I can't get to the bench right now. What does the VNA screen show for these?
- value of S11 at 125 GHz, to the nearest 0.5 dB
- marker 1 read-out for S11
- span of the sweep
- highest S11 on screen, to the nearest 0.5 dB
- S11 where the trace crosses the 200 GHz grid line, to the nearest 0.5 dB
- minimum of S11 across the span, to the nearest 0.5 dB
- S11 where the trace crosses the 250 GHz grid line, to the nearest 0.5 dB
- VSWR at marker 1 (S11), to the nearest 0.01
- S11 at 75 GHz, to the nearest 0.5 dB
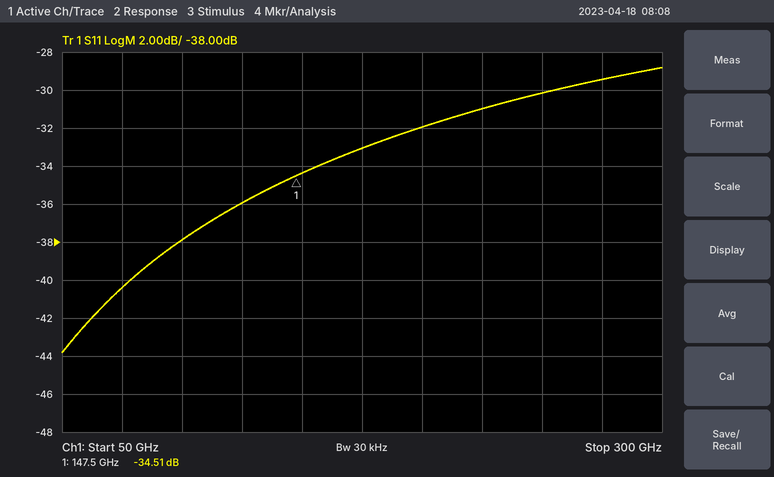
-36.0 dB
-34.51 dB
250 GHz
-29.0 dB
-32.0 dB
-44.0 dB
-30.0 dB
1.04
-40.5 dB
